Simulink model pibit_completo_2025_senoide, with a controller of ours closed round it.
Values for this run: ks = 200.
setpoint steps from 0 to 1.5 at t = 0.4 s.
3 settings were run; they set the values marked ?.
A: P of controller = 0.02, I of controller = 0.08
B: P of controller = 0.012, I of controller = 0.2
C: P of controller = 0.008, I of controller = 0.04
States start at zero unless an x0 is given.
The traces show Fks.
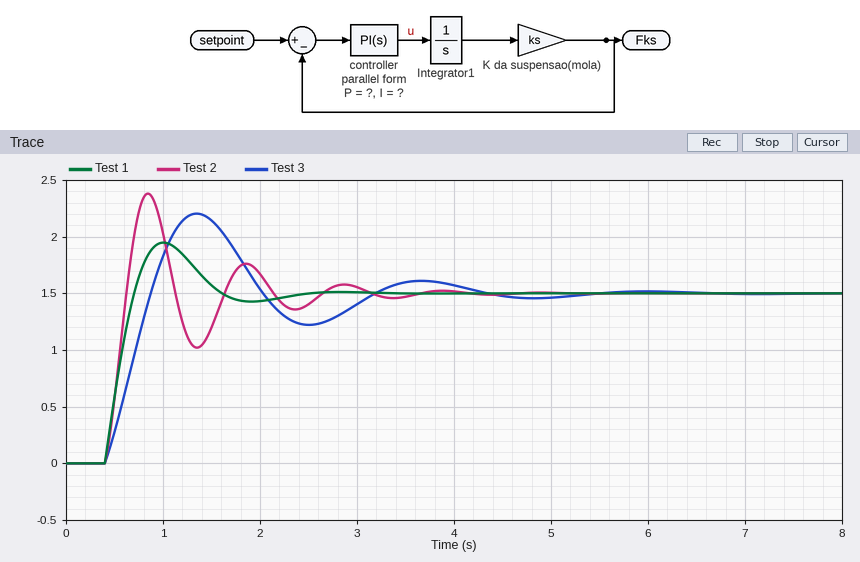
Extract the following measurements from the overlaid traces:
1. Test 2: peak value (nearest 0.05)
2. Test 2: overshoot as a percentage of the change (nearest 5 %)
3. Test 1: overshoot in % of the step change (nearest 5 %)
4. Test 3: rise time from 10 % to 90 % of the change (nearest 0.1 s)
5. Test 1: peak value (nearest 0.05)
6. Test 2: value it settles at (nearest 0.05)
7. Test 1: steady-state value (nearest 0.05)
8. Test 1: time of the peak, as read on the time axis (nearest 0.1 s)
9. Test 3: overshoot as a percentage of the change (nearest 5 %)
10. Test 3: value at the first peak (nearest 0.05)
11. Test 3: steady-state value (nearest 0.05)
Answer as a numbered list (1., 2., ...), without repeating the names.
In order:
1. 2.40
2. 60 %
3. 30 %
4. 0.4 s
5. 1.95
6. 1.50
7. 1.50
8. 1.0 s
9. 45 %
10. 2.20
11. 1.50
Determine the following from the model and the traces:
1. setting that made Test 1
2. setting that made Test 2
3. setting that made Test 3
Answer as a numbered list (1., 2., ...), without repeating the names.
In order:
1. A
2. B
3. C
